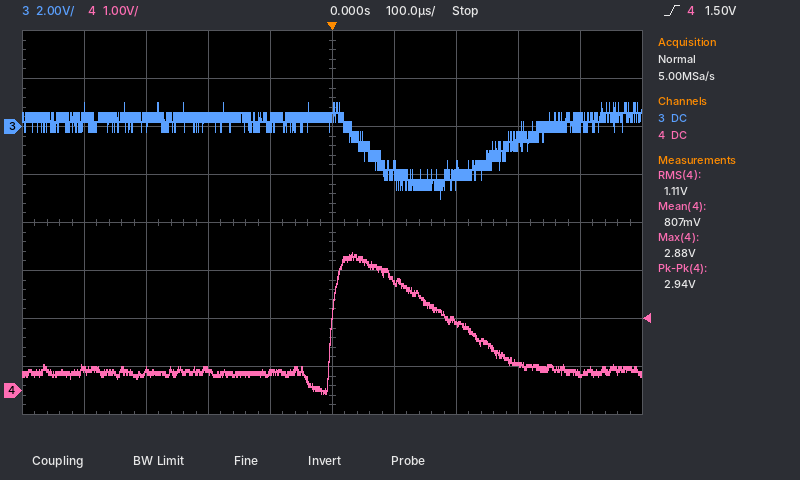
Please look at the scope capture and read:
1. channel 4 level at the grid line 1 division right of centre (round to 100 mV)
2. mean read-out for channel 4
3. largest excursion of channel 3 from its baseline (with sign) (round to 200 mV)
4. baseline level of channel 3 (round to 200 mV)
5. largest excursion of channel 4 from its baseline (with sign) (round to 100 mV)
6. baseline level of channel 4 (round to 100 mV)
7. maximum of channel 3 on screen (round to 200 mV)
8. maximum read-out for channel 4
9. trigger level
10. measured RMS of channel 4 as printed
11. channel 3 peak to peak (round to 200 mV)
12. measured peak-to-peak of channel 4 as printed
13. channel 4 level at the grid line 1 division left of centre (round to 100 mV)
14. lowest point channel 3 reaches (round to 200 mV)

2.3 V
807 mV
-3.4 V
400 mV
+2.5 V
400 mV
1.0 V
2.88 V
1.50 V
1.11 V
4.0 V
2.94 V
400 mV
-3.0 V
